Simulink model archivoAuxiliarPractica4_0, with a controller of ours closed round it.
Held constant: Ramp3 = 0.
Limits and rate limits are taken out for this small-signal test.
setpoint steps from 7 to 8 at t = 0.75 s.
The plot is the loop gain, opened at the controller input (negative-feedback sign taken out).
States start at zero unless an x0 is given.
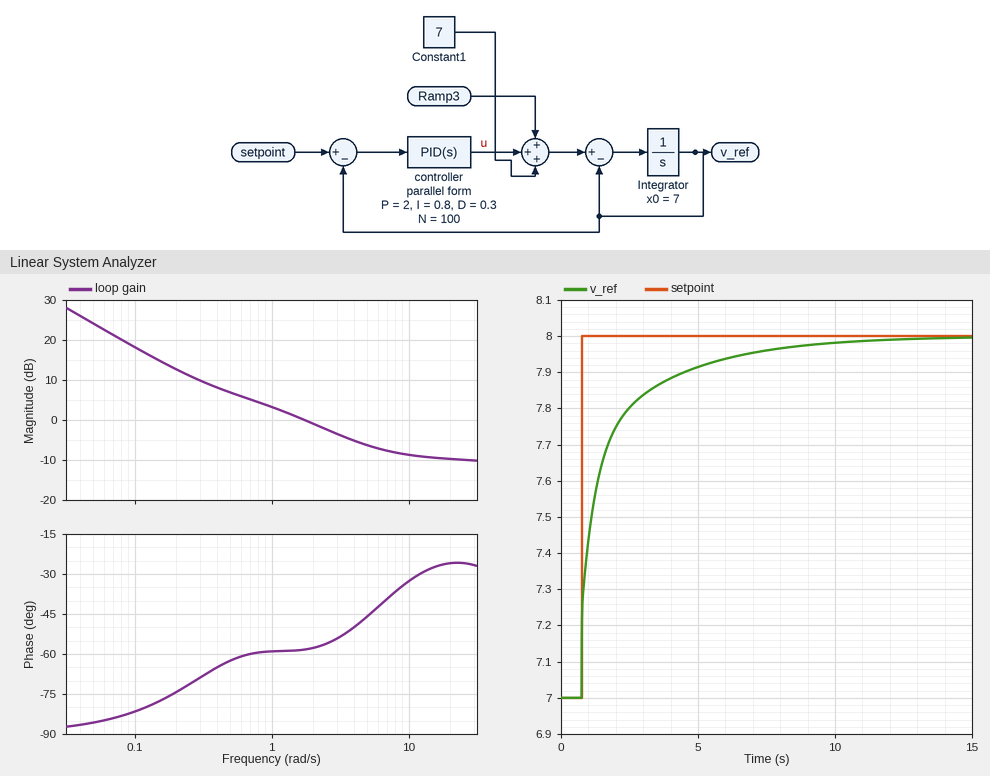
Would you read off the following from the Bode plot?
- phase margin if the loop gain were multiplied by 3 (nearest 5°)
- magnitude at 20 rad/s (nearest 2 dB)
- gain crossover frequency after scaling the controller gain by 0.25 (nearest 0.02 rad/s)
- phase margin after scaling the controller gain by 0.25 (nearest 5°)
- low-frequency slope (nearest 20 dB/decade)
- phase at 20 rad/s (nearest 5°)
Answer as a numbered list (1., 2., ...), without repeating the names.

1. 155°
2. -10 dB
3. 0.22 rad/s
4. 105°
5. -20 dB/decade
6. -25°
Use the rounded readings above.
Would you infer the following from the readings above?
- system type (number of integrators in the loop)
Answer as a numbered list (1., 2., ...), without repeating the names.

1. 1
